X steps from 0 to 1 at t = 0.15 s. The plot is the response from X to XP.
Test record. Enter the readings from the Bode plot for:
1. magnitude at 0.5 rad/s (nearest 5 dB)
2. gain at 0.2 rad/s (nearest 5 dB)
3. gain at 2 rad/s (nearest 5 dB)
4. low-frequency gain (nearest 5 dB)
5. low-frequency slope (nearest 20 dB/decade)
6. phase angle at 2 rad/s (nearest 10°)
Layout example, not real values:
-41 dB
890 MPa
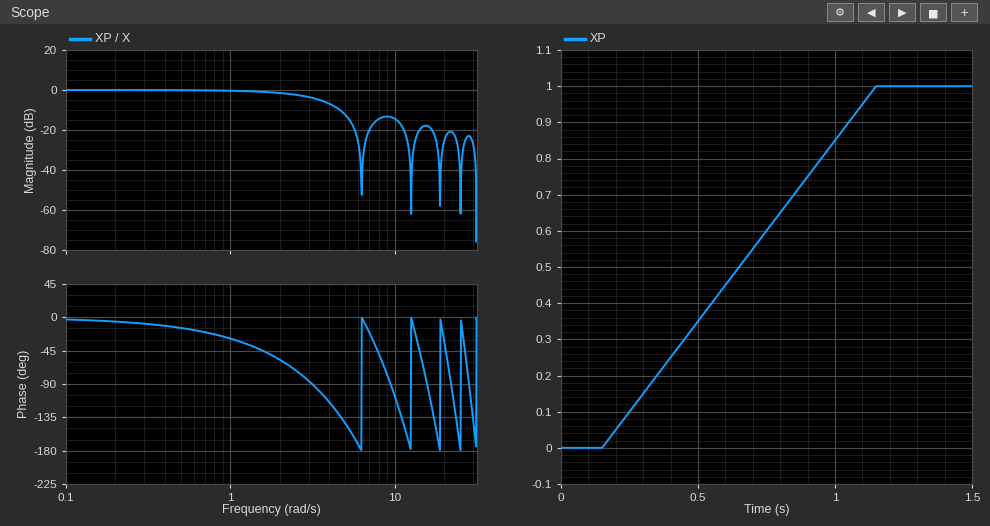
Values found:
0 dB
0 dB
0 dB
0 dB
0 dB/decade
-60°
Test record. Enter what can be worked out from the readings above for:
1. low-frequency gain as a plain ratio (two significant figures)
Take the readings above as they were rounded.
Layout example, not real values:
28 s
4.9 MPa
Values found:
1.0
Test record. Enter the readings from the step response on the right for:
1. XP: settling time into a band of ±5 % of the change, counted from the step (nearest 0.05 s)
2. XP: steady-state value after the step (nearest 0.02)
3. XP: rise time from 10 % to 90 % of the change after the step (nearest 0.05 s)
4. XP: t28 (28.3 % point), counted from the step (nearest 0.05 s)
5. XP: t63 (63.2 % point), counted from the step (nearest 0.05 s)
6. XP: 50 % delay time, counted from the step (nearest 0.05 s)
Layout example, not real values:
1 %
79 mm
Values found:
0.95 s
1.00
0.80 s
0.30 s
0.65 s
0.50 s
